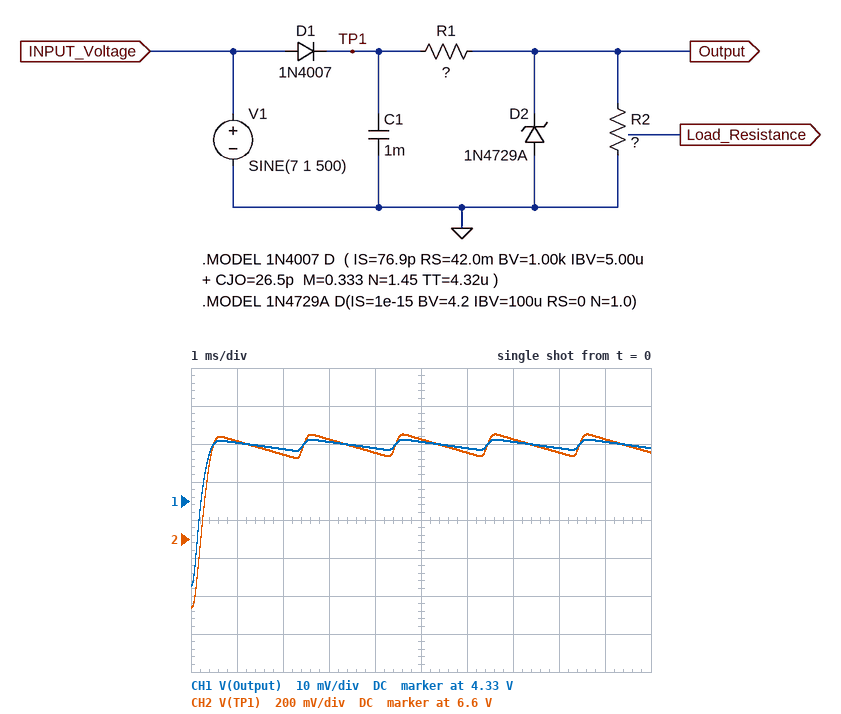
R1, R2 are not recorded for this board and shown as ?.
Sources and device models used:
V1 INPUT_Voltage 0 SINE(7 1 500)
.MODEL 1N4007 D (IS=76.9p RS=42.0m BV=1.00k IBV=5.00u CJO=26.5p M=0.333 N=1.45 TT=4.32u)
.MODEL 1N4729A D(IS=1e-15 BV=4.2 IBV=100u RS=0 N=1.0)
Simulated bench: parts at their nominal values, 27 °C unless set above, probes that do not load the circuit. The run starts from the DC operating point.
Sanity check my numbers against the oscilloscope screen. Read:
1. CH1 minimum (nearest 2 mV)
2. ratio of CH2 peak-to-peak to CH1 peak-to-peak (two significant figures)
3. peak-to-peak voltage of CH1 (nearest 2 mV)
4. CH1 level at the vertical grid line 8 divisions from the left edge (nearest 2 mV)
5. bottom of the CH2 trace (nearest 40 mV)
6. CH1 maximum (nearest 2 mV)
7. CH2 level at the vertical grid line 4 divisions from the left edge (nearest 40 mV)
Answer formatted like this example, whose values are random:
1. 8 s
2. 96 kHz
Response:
1. 4.308 V
2. 24
3. 38 mV
4. 4.344 V
5. 6.24 V
6. 4.346 V
7. 7.04 V
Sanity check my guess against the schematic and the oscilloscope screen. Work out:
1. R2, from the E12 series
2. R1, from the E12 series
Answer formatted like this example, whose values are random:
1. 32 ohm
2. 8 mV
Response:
1. 100 Ω
2. 39 Ω
